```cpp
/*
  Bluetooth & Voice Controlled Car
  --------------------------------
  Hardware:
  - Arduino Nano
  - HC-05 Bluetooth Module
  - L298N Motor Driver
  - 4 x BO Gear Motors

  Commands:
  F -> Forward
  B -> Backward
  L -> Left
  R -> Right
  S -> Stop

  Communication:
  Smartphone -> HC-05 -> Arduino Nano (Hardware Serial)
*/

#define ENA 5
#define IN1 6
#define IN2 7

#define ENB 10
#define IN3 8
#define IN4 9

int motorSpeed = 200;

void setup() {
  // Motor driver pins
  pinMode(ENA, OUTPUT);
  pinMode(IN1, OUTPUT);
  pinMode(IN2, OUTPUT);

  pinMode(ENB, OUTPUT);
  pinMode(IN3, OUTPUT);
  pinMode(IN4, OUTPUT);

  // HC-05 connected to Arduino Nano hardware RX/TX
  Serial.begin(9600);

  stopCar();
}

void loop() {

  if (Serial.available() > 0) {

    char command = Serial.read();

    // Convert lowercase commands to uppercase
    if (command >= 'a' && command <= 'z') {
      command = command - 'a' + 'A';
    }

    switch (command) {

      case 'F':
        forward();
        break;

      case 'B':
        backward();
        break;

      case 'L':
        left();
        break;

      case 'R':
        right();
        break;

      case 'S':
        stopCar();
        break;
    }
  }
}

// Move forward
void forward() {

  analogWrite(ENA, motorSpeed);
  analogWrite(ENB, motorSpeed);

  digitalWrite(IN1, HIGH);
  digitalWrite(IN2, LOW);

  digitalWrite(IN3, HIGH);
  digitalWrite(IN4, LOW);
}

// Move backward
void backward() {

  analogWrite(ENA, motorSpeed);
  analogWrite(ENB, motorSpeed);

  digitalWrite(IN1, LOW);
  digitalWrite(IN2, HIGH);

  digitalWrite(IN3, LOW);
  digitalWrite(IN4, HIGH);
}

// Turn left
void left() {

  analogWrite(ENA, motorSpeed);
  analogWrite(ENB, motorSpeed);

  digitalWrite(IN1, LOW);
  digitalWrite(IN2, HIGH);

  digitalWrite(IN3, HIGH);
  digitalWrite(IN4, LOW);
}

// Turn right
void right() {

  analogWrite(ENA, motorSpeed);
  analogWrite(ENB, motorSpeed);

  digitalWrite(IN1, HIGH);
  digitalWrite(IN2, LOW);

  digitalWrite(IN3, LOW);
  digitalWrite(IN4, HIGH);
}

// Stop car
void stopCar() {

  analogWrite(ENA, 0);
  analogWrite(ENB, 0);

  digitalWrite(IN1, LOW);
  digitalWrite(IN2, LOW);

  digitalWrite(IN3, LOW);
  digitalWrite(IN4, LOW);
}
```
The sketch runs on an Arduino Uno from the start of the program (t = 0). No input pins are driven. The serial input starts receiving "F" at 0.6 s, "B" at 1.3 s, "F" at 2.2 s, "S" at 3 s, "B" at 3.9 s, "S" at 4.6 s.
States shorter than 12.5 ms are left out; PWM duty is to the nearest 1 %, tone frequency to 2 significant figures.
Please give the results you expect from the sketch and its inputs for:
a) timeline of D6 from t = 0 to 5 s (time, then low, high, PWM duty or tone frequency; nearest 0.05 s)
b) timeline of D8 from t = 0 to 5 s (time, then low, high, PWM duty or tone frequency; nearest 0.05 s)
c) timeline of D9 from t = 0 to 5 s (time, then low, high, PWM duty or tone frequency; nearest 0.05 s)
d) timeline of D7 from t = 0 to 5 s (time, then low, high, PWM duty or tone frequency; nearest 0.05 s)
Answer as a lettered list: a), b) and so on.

a) 0 s low; 0.6 s high; 1.3 s low; 2.2 s high; 3 s low
b) 0 s low; 0.6 s high; 1.3 s low; 2.2 s high; 3 s low
c) 0 s low; 1.3 s high; 2.2 s low; 3.9 s high; 4.6 s low
d) 0 s low; 1.3 s high; 2.2 s low; 3.9 s high; 4.6 s low
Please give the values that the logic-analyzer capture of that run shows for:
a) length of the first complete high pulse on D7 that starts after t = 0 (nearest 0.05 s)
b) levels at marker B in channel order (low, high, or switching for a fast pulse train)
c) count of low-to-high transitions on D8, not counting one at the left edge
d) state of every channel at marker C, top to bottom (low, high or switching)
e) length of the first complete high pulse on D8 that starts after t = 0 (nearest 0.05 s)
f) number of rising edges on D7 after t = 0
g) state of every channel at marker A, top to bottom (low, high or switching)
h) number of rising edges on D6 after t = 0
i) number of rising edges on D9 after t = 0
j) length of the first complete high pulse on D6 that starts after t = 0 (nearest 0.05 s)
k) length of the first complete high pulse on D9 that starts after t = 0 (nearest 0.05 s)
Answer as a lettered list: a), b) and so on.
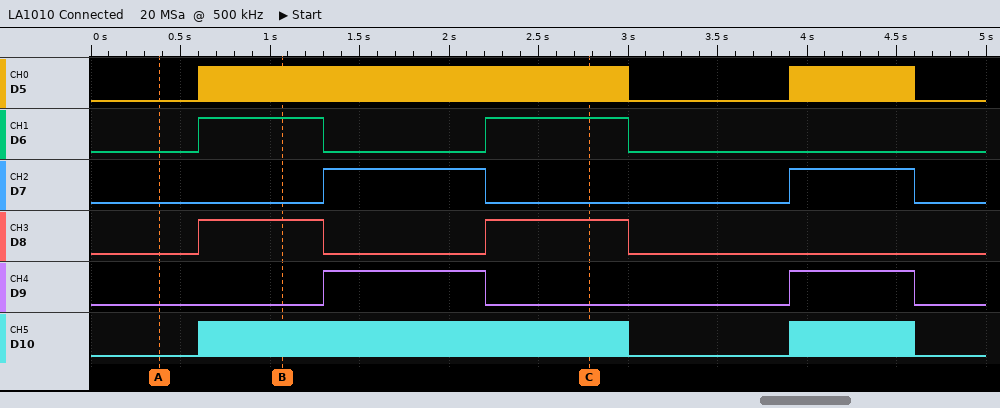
a) 0.90 s
b) D5 switching, D6 high, D7 low, D8 high, D9 low, D10 switching
c) 2
d) D5 switching, D6 high, D7 low, D8 high, D9 low, D10 switching
e) 0.70 s
f) 2
g) D5 low, D6 low, D7 low, D8 low, D9 low, D10 low
h) 2
i) 2
j) 0.70 s
k) 0.90 s
